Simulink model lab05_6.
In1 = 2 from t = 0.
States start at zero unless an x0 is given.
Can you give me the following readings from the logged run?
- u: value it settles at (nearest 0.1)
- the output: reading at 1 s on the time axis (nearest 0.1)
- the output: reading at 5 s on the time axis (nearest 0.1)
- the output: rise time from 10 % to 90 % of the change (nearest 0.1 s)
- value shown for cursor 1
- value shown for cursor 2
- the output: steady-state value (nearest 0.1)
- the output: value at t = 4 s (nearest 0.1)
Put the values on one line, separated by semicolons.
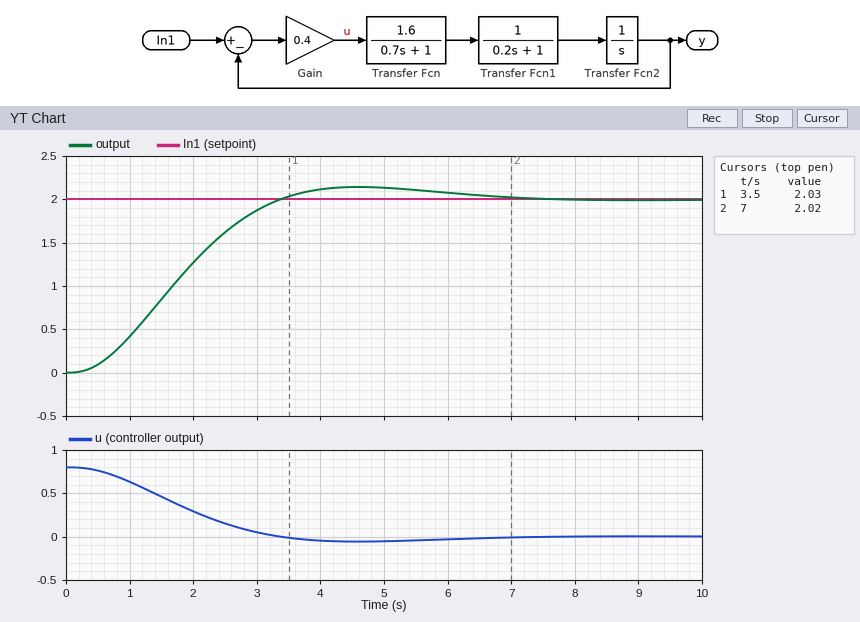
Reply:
0.0; 0.4; 2.1; 2.1 s; 2.03; 2.02; 2.0; 2.1
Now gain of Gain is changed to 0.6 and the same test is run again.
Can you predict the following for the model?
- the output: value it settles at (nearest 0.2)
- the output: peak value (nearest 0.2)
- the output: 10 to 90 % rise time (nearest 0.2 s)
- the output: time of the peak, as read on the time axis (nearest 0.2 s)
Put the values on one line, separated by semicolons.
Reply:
2.0; 2.4; 1.4 s; 3.4 s
